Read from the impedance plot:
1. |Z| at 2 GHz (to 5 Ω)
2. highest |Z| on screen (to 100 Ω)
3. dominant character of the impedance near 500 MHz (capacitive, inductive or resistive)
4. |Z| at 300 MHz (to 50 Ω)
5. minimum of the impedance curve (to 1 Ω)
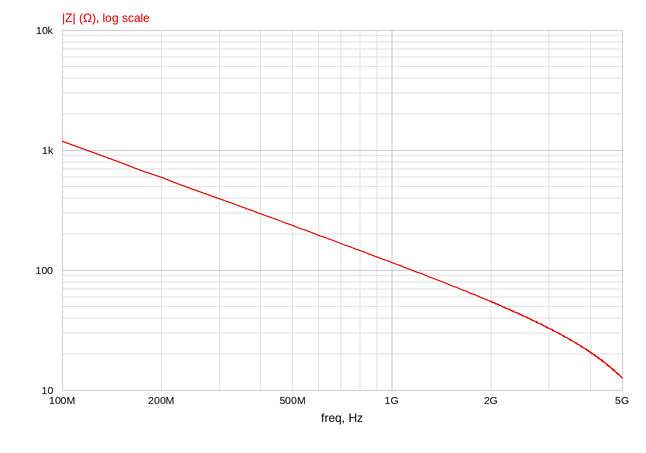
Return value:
55 Ω
1.2 kΩ
capacitive
400 Ω
13 Ω
